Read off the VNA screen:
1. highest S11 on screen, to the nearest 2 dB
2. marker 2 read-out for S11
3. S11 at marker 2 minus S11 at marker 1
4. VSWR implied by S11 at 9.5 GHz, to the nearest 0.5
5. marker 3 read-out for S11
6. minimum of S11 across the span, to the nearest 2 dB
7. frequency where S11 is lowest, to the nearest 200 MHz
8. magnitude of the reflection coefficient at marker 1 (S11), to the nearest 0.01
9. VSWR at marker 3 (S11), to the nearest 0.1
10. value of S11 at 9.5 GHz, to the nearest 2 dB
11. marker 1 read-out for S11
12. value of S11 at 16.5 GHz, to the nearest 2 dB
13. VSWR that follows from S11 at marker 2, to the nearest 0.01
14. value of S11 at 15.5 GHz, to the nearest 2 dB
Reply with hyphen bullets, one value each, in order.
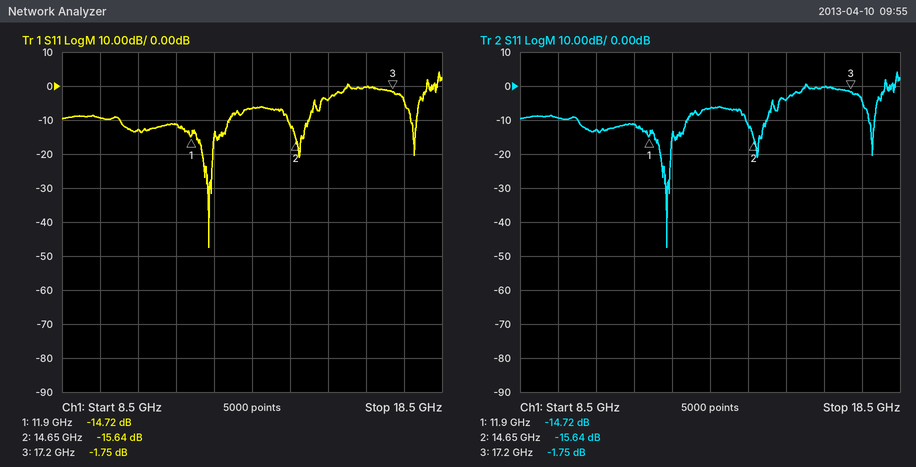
- 4 dB
- -15.64 dB
- -0.92 dB
- 2.0
- -1.75 dB
- -48 dB
- 12.4 GHz
- 0.18
- 10.0
- -10 dB
- -14.72 dB
- 0 dB
- 1.40
- -4 dB
